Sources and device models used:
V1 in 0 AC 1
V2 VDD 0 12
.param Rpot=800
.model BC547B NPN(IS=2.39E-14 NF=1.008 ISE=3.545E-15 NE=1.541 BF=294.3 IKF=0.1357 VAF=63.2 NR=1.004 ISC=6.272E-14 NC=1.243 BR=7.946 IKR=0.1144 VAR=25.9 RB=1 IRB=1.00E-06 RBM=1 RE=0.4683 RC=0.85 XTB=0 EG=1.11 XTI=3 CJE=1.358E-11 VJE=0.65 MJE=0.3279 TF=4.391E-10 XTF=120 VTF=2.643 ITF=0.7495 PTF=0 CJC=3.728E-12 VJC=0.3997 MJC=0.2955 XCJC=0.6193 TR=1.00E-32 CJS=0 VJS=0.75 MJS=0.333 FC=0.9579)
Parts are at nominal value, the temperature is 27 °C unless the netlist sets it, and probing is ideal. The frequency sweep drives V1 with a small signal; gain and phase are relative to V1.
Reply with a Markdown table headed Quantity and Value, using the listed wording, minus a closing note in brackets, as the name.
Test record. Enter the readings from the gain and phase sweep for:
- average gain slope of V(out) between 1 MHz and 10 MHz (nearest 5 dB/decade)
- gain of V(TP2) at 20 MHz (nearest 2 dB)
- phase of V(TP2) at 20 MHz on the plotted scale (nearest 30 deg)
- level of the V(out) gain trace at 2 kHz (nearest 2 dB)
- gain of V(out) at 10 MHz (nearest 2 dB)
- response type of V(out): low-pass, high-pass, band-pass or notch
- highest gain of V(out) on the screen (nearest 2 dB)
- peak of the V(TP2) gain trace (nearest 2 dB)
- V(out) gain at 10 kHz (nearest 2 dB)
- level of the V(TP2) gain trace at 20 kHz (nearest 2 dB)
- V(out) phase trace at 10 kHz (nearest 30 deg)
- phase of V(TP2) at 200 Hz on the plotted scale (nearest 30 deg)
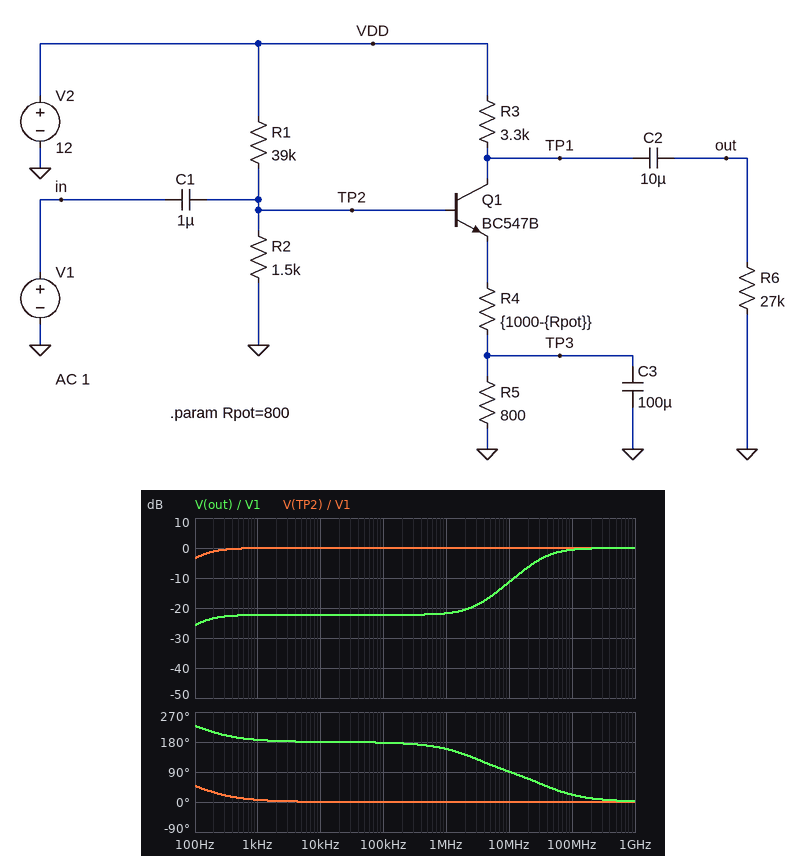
| Quantity | Value |
|---|---|
| average gain slope of V(out) between 1 MHz and 10 MHz | 10 dB/decade |
| gain of V(TP2) at 20 MHz | 0 dB |
| phase of V(TP2) at 20 MHz on the plotted scale | 0 deg |
| level of the V(out) gain trace at 2 kHz | -22 dB |
| gain of V(out) at 10 MHz | -12 dB |
| response type of V(out): low-pass, high-pass, band-pass or notch | high-pass |
| highest gain of V(out) on the screen | 0 dB |
| peak of the V(TP2) gain trace | 0 dB |
| V(out) gain at 10 kHz | -22 dB |
| level of the V(TP2) gain trace at 20 kHz | 0 dB |
| V(out) phase trace at 10 kHz | 180 deg |
| phase of V(TP2) at 200 Hz on the plotted scale | 30 deg |
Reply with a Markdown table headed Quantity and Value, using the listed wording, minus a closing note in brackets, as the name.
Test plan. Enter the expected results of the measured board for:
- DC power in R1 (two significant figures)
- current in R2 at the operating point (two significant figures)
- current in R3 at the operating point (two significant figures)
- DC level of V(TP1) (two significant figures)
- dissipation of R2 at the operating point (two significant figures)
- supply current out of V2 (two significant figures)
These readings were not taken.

| Quantity | Value |
|---|---|
| DC power in R1 | 3.4 mW |
| current in R2 at the operating point | 300 µA |
| current in R3 at the operating point | 690 nA |
| DC level of V(TP1) | 12 V |
| dissipation of R2 at the operating point | 130 µW |
| supply current out of V2 | 300 µA |
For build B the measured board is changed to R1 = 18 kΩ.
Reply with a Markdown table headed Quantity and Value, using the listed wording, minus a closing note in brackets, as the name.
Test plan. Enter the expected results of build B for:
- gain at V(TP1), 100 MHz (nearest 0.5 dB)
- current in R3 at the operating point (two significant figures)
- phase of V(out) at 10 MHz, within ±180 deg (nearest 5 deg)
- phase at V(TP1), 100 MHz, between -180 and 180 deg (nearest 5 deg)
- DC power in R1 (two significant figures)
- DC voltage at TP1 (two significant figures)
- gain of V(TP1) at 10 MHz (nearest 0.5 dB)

| Quantity | Value |
|---|---|
| gain at V(TP1), 100 MHz | 9.5 dB |
| current in R3 at the operating point | 320 µA |
| phase of V(out) at 10 MHz, within ±180 deg | 155 deg |
| phase at V(TP1), 100 MHz, between -180 and 180 deg | 45 deg |
| DC power in R1 | 6.8 mW |
| DC voltage at TP1 | 11 V |
| gain of V(TP1) at 10 MHz | 20.0 dB |
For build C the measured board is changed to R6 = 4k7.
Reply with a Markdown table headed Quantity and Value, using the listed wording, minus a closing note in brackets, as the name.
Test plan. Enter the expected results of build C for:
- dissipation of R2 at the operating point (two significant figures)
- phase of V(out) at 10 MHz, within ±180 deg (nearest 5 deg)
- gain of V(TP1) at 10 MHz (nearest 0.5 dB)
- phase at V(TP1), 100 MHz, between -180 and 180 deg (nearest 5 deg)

| Quantity | Value |
|---|---|
| dissipation of R2 at the operating point | 130 µW |
| phase of V(out) at 10 MHz, within ±180 deg | 95 deg |
| gain of V(TP1) at 10 MHz | -15.0 dB |
| phase at V(TP1), 100 MHz, between -180 and 180 deg | 30 deg |
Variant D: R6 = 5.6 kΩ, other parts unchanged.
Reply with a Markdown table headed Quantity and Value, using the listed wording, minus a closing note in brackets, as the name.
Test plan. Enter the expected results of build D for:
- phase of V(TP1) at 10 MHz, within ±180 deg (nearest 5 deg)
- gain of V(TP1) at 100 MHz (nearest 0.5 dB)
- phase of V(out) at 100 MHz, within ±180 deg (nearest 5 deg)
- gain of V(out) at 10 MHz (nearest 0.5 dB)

| Quantity | Value |
|---|---|
| phase of V(TP1) at 10 MHz, within ±180 deg | 95 deg |
| gain of V(TP1) at 100 MHz | -1.0 dB |
| phase of V(out) at 100 MHz, within ±180 deg | 30 deg |
| gain of V(out) at 10 MHz | -14.0 dB |
